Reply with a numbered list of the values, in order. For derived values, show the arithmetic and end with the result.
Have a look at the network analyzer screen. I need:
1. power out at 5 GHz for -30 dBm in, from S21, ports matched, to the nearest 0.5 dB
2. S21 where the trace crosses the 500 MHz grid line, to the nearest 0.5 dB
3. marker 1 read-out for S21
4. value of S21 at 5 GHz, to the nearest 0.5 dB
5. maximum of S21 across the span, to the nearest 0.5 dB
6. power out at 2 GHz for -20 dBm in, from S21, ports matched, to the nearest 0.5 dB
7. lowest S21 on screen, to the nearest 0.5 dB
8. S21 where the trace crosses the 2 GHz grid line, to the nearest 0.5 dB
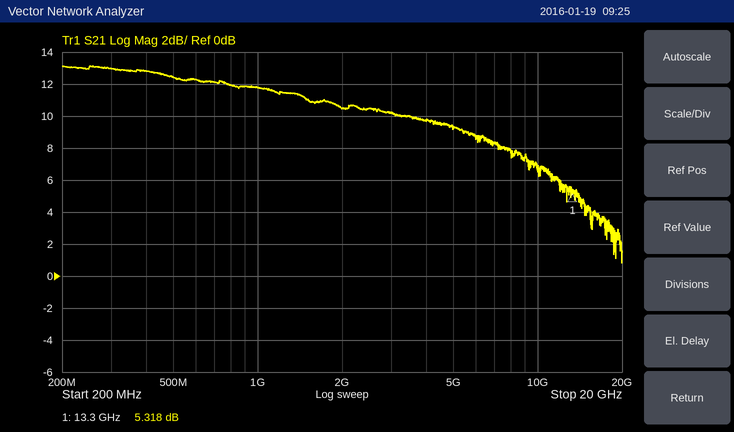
1. -30 dBm + (9.5 dB) = -20.5 dBm
2. 12.5 dB
3. 5.318 dB
4. 9.5 dB
5. 13.0 dB
6. -20 dBm + (10.5 dB) = -9.5 dBm
7. 1.0 dB
8. 10.5 dB
